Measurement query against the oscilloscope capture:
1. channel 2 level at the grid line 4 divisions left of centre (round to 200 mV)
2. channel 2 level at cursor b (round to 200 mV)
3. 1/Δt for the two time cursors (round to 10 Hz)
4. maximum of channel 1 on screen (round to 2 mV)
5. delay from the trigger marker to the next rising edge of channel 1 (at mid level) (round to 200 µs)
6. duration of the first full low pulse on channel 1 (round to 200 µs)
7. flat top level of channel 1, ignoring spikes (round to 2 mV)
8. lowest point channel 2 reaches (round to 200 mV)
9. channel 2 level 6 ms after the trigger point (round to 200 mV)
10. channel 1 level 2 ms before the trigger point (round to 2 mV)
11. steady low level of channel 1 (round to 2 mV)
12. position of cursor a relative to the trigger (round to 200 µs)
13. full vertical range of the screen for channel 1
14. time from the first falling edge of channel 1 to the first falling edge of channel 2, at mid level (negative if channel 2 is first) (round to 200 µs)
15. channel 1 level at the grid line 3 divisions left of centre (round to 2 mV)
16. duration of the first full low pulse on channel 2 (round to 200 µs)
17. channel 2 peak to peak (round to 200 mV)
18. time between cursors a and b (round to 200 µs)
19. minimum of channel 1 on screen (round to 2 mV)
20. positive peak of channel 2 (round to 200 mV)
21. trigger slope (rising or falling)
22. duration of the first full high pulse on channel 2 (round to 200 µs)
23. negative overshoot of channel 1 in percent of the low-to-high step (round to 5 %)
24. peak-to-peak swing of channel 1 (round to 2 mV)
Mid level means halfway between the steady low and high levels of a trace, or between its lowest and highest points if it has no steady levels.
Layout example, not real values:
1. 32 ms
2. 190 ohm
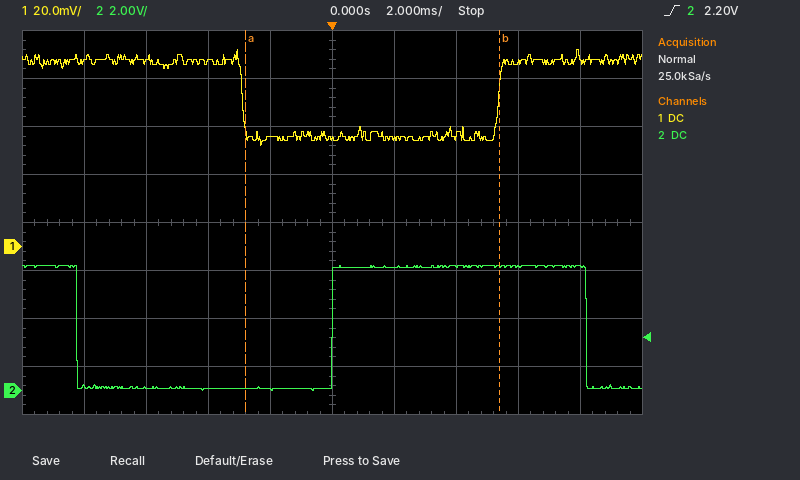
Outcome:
1. 200 mV
2. 5.2 V
3. 120 Hz
4. 82 mV
5. 5.4 ms
6. 8.2 ms
7. 78 mV
8. 0.0 V
9. 5.2 V
10. 46 mV
11. 46 mV
12. -2.8 ms
13. 160 mV
14. -5.4 ms
15. 78 mV
16. 8.2 ms
17. 5.2 V
18. 8.2 ms
19. 42 mV
20. 5.2 V
21. rising
22. 8.2 ms
23. 10 %
24. 40 mV
